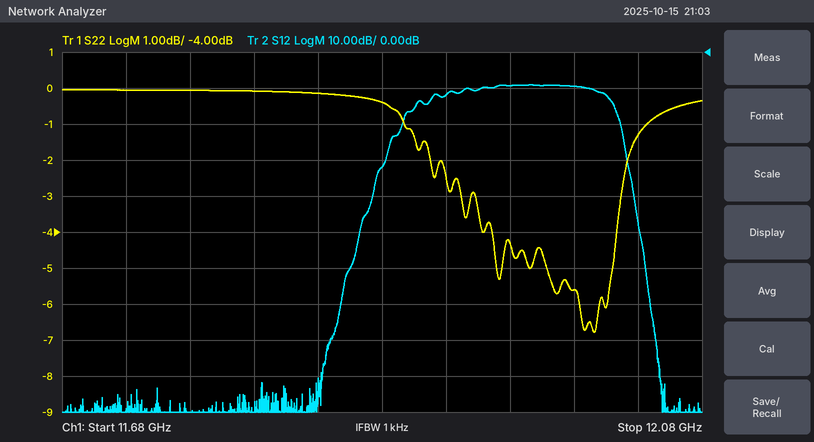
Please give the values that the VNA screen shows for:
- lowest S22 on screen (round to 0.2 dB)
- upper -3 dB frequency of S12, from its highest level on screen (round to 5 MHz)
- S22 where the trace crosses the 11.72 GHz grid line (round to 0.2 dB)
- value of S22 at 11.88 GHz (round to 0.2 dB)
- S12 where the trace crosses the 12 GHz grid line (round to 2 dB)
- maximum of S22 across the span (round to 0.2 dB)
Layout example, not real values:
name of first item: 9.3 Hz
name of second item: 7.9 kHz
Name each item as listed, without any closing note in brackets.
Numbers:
lowest S22 on screen: -6.8 dB
upper -3 dB frequency of S12, from its highest level on screen: 12.020 GHz
S22 where the trace crosses the 11.72 GHz grid line: 0.0 dB
value of S22 at 11.88 GHz: -0.4 dB
S12 where the trace crosses the 12 GHz grid line: -10 dB
maximum of S22 across the span: 0.0 dB
